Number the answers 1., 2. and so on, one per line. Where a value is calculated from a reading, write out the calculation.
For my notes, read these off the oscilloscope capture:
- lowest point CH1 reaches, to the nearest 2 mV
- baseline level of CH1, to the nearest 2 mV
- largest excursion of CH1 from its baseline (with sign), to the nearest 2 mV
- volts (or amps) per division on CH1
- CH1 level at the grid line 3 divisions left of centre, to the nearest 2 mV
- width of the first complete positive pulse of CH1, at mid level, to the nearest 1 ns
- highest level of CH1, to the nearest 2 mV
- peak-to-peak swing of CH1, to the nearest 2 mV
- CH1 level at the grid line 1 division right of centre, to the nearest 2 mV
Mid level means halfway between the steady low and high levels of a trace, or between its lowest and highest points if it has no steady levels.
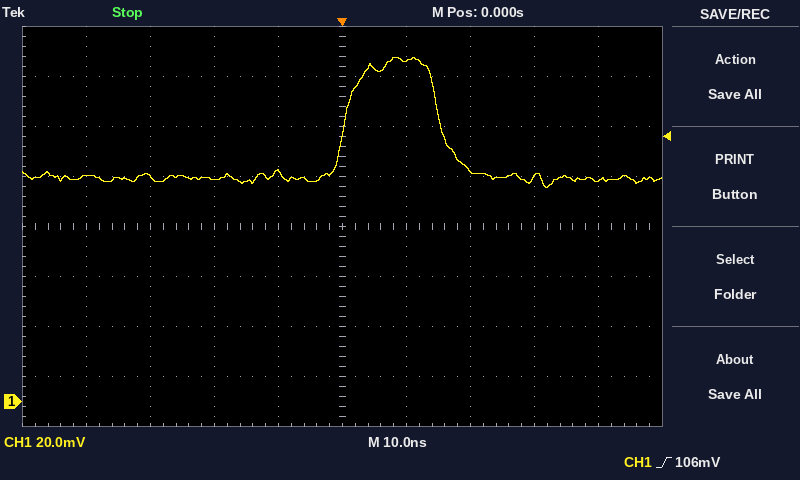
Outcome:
1. 86 mV
2. 90 mV
3. 138 mV − (90 mV) = +48 mV
4. 20 mV
5. 90 mV
6. 15 ns
7. 138 mV
8. 138 mV − (86 mV) = 52 mV
9. 136 mV
